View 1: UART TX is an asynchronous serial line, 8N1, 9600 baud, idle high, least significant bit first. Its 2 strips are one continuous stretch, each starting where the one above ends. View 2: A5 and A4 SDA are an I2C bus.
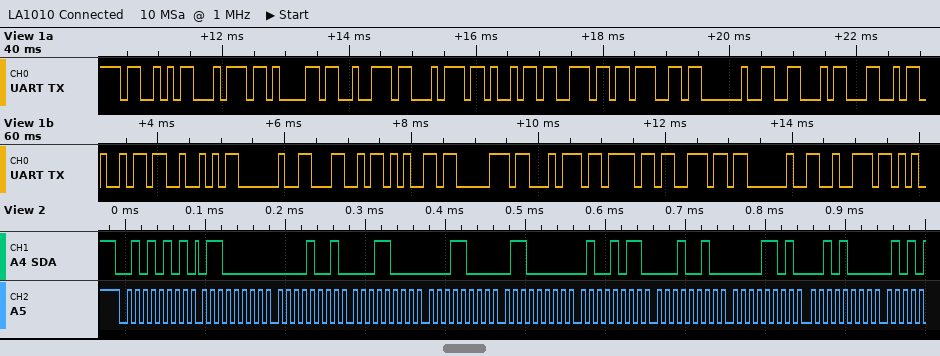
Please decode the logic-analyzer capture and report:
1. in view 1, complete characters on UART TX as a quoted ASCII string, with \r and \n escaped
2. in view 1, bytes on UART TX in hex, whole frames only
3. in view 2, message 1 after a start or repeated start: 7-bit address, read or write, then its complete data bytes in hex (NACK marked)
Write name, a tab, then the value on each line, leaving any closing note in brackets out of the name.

in view 1, complete characters on UART TX as a quoted ASCII string, with \r and \n escaped	"Starting FLiR Lepton r"
in view 1, bytes on UART TX in hex, whole frames only	53 74 61 72 74 69 6E 67 20 46 4C 69 52 20 4C 65 70 74 6F 6E 20 72
in view 2, message 1 after a start or repeated start: 7-bit address, read or write, then its complete data bytes in hex	0x2A read: 60 09 18 18 60 4B 12 0D 28
